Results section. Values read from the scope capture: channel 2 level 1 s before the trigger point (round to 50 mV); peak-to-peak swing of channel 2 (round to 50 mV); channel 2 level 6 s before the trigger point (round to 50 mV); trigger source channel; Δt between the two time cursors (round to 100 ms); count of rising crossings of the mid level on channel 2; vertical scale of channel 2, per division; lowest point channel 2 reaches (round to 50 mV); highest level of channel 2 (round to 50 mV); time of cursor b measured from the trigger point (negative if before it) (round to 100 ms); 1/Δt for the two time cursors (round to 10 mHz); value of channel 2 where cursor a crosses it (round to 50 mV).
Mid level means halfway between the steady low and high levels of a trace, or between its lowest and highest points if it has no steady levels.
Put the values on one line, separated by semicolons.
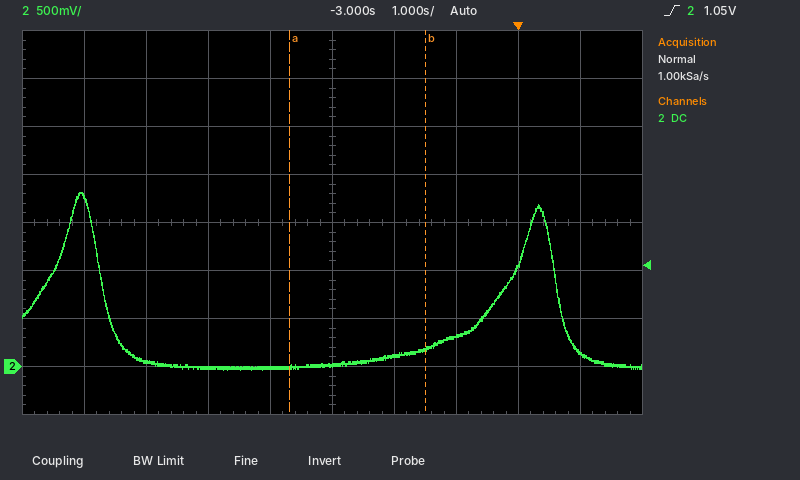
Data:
300 mV; 1.85 V; 50 mV; channel 2; 2.2 s; 2; 500 mV; -50 mV; 1.80 V; -1.5 s; 450 mHz; 0 mV
